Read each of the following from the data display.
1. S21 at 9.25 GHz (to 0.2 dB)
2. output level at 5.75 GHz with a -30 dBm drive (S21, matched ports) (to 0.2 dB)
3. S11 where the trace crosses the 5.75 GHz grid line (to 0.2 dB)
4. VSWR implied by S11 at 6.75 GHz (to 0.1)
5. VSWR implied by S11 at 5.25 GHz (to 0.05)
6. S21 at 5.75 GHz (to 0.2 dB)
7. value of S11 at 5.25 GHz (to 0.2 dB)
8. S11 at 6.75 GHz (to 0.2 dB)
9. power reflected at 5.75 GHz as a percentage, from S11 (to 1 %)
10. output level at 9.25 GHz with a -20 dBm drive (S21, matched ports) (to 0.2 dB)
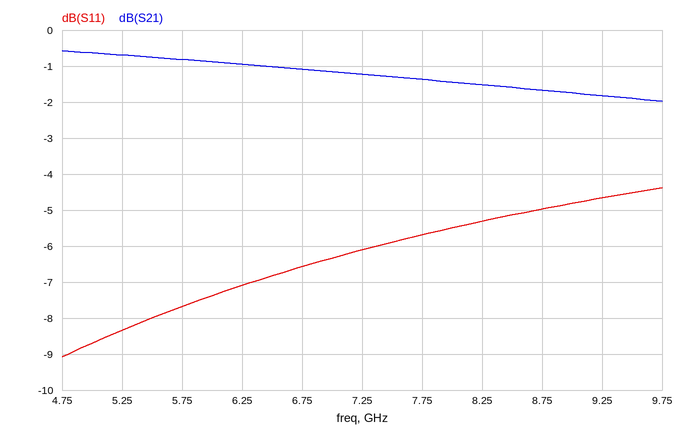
-1.8 dB
-30.8 dBm
-7.6 dB
2.8
2.25
-0.8 dB
-8.4 dB
-6.6 dB
17 %
-21.8 dBm
